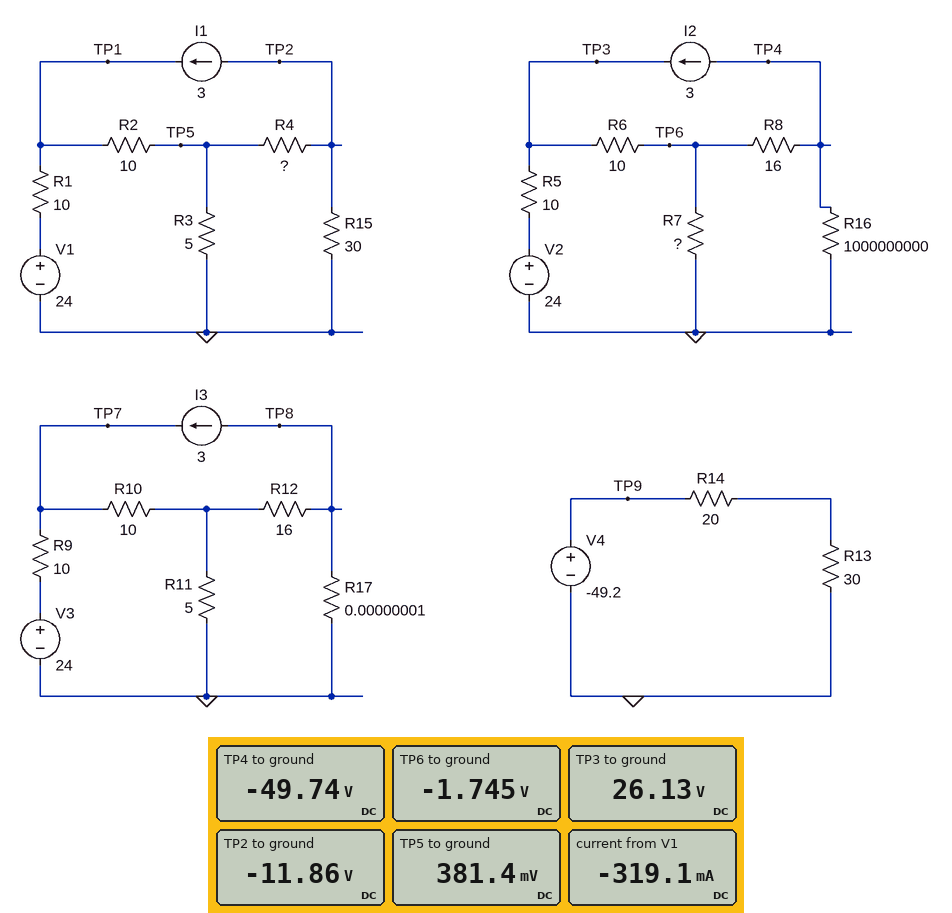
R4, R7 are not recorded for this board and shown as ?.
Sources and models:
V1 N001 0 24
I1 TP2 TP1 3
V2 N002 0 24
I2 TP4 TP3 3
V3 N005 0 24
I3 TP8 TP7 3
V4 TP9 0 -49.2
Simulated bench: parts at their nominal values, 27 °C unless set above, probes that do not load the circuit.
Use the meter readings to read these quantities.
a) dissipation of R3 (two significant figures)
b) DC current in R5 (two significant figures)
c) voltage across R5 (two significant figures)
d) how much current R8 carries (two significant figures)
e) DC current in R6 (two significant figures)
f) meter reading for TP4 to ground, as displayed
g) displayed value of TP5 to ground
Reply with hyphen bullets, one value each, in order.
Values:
- 29 mW
- 210 mA
- 2.1 V
- 3.0 A
- 2.8 A
- -49.74 V
- 381.4 mV
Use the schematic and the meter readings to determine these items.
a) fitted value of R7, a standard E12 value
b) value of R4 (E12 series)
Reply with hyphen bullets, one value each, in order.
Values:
- 8.2 Ω
- 4.7 Ω
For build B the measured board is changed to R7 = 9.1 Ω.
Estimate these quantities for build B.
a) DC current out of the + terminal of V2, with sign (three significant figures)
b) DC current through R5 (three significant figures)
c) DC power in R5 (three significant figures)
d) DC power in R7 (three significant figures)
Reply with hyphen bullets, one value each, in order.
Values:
- -206 mA
- 206 mA
- 425 mW
- 387 mW
